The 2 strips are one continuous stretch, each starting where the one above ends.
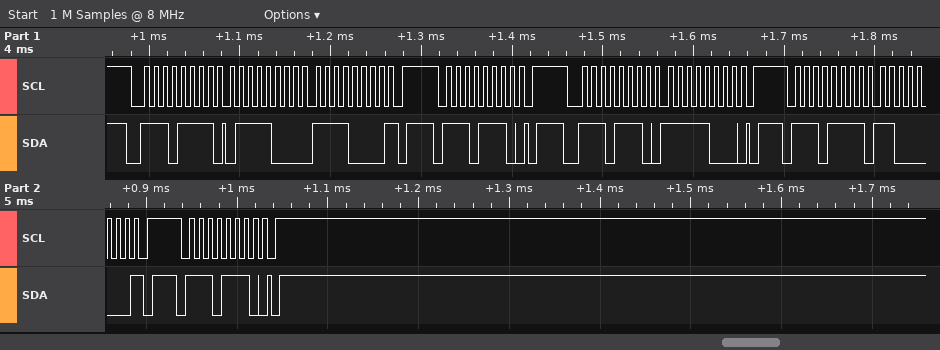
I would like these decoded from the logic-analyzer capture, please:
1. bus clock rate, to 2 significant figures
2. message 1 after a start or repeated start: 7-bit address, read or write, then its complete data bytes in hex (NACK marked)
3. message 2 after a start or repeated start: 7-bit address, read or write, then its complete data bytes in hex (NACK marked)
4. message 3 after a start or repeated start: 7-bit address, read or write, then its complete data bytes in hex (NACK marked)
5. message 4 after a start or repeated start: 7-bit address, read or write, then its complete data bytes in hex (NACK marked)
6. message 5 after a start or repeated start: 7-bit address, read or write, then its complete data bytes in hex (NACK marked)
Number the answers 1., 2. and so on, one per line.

1. 100 kHz
2. 0x77 read: 78 F0 NACK
3. 0x77 write
4. 0x77 write: F8
5. 0x77 read: C0 NACK
6. 0x77 write
